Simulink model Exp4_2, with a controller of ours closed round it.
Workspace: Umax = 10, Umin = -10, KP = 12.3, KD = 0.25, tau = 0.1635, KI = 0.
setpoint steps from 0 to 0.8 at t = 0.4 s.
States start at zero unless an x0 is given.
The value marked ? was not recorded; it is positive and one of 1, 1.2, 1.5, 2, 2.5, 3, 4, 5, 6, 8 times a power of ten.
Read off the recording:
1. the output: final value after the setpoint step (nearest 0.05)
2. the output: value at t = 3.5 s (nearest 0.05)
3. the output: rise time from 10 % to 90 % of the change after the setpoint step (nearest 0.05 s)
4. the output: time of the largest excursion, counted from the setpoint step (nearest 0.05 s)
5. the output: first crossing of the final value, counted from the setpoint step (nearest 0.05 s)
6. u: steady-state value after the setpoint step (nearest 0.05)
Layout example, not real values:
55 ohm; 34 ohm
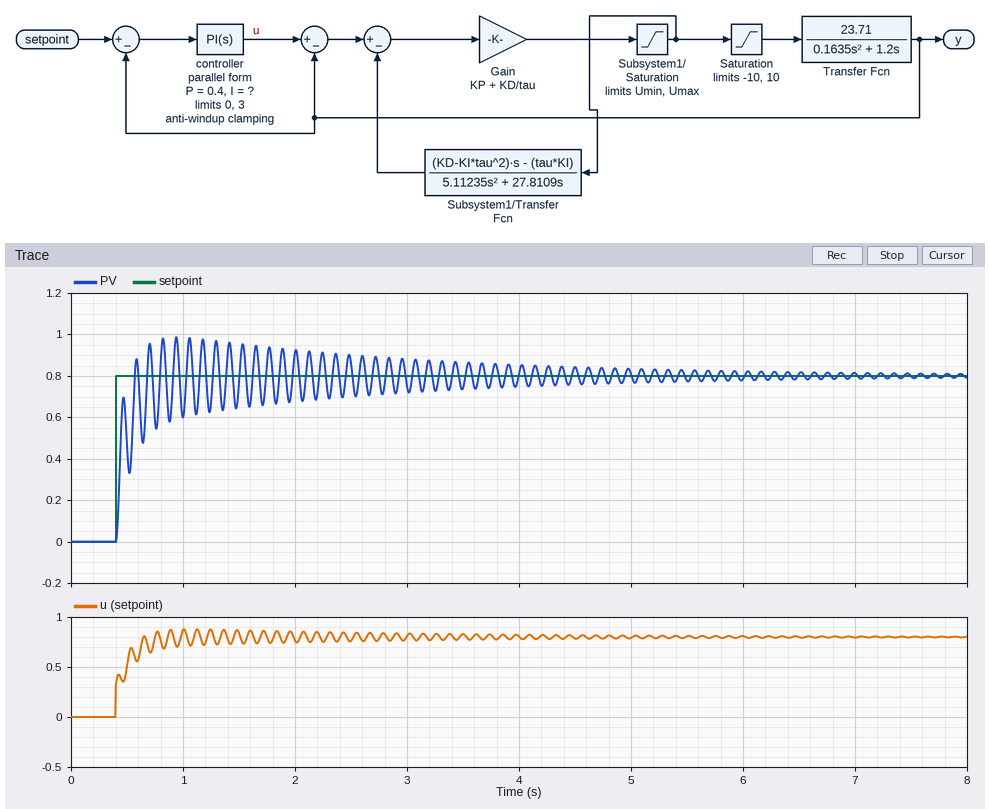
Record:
0.80; 0.75; 0.15 s; 0.55 s; 0.15 s; 0.80
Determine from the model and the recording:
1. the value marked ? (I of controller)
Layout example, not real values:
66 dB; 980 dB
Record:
10
